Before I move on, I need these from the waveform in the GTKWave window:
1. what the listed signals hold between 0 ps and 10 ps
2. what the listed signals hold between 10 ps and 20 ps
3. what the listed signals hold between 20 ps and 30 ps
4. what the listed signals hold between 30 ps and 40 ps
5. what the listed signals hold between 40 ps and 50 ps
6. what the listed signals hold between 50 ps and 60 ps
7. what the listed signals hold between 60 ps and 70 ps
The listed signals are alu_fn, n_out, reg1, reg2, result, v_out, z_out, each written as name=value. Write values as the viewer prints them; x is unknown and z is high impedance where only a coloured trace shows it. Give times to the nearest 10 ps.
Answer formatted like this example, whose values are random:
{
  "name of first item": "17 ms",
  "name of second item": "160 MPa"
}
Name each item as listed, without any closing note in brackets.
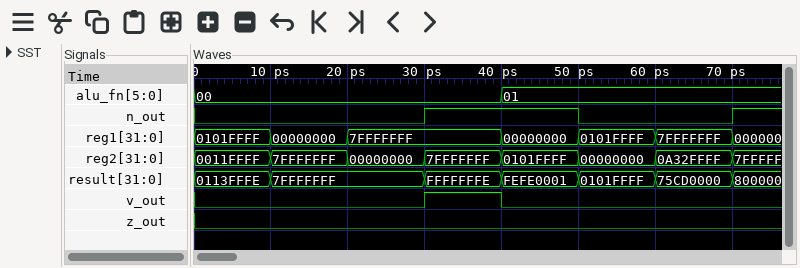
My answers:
{
  "what the listed signals hold between 0 ps and 10 ps": "alu_fn=00, n_out=0, reg1=0101FFFF, reg2=0011FFFF, result=0113FFFE, v_out=0, z_out=0",
  "what the listed signals hold between 10 ps and 20 ps": "alu_fn=00, n_out=0, reg1=00000000, reg2=7FFFFFFF, result=7FFFFFFF, v_out=0, z_out=0",
  "what the listed signals hold between 20 ps and 30 ps": "alu_fn=00, n_out=0, reg1=7FFFFFFF, reg2=00000000, result=7FFFFFFF, v_out=0, z_out=0",
  "what the listed signals hold between 30 ps and 40 ps": "alu_fn=00, n_out=1, reg1=7FFFFFFF, reg2=7FFFFFFF, result=FFFFFFFE, v_out=1, z_out=0",
  "what the listed signals hold between 40 ps and 50 ps": "alu_fn=01, n_out=1, reg1=00000000, reg2=0101FFFF, result=FEFE0001, v_out=0, z_out=0",
  "what the listed signals hold between 50 ps and 60 ps": "alu_fn=01, n_out=0, reg1=0101FFFF, reg2=00000000, result=0101FFFF, v_out=0, z_out=0",
  "what the listed signals hold between 60 ps and 70 ps": "alu_fn=01, n_out=0, reg1=7FFFFFFF, reg2=0A32FFFF, result=75CD0000, v_out=0, z_out=0"
}
